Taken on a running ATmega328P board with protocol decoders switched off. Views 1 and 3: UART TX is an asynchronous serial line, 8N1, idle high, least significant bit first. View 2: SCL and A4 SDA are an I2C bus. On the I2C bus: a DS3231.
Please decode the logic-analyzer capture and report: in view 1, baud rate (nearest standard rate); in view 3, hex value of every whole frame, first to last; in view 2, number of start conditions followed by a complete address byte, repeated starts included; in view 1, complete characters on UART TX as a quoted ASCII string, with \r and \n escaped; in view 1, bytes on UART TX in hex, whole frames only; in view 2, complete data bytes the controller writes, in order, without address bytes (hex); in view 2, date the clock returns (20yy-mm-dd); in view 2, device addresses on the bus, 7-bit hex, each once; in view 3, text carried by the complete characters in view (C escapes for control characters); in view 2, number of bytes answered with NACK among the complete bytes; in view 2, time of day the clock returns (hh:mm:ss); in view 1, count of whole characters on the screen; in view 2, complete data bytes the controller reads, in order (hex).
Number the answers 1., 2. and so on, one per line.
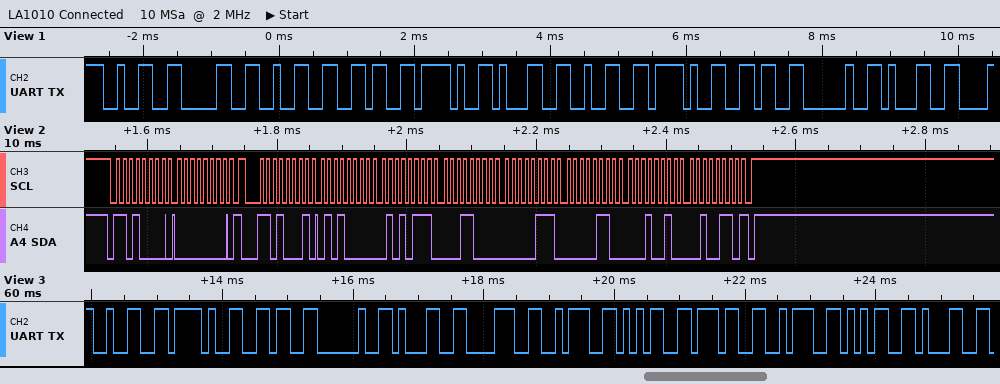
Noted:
1. 9600 baud
2. 0x32 0x2F 0x36 0x20 0x31 0x38 0x3A 0x35 0x37 0x3A 0x35 0x31
3. 2
4. "2026/12/6 1"
5. 32 30 32 36 2F 31 32 2F 36 20 31
6. 00
7. 2026-12-06
8. 0x68
9. "2/6 18:57:51"
10. 1
11. 18:57:50
12. 11
13. 50 57 18 07 06 12 26
